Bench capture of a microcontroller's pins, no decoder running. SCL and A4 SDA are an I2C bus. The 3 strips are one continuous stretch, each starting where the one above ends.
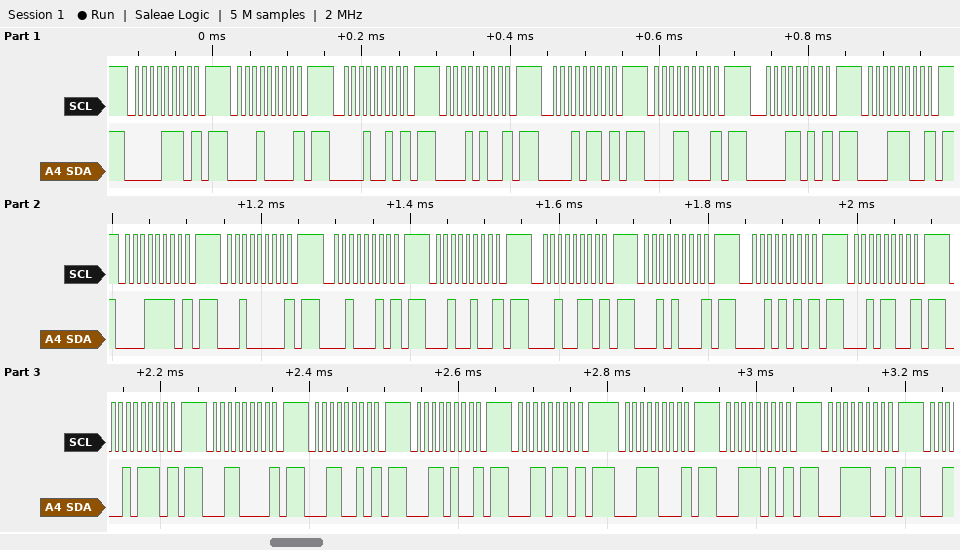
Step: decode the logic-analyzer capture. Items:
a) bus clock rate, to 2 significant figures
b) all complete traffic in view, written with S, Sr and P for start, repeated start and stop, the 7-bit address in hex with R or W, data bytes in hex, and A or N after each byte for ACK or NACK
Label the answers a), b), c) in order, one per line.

a) 100 kHz
b) S 07W N P S 08W N P S 09W N P S 0AW N P S 0BW N P S 0CW N P S 0DW N P S 0EW N P S 0FW N P S 10W N P S 11W N P S 12W N P S 13W N P S 14W N P S 15W N P S 16W N P S 17W N P S 18W N P S 19W N P S 1AW N P S 1BW N P S 1CW N P S 1DW N P S 1EW N P
